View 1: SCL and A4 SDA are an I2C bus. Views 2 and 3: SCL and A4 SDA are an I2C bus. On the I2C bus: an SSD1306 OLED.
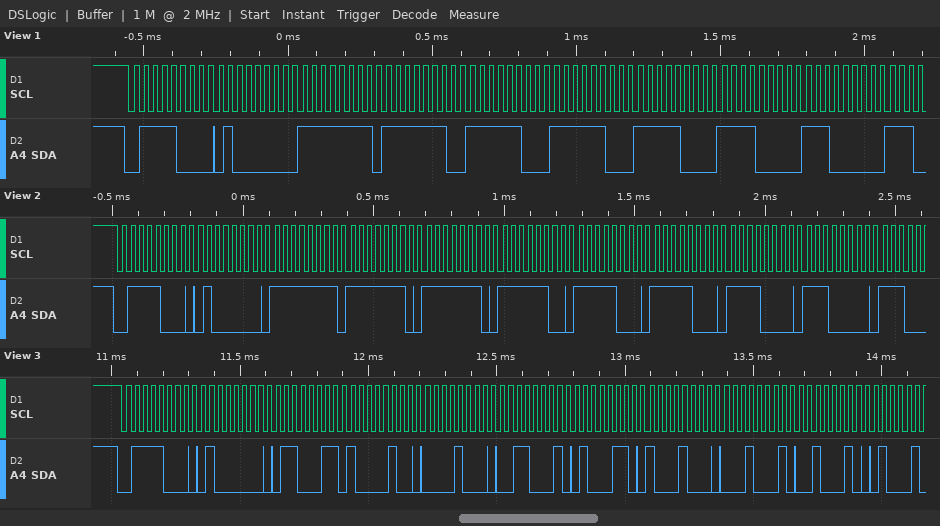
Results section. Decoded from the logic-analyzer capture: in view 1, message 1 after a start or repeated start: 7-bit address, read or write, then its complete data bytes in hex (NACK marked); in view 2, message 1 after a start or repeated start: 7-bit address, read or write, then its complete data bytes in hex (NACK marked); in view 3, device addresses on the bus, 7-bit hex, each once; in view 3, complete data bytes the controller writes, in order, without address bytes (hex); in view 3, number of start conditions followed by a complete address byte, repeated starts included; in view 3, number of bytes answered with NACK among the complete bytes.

0x3C write: 40 FF FE FC FC F8 F0 E0
0x3C write: 40 FF FE FE FC F8 F8 F0 E0
0x3C
40 63 84 08 31 46 88 11 22
1
0
